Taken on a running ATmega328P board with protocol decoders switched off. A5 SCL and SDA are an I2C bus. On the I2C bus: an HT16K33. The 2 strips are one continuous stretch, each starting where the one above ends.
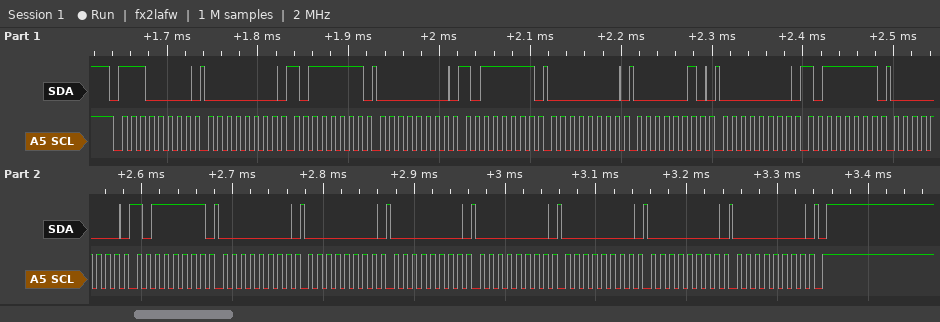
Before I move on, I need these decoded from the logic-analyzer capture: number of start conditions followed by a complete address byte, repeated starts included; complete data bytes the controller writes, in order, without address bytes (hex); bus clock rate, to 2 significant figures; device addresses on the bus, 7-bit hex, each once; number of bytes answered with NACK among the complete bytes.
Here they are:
1
00 BF 00 BF 00 02 00 BF 00 BF 00 00 00 00 00 00 00
100 kHz
0x70
0
